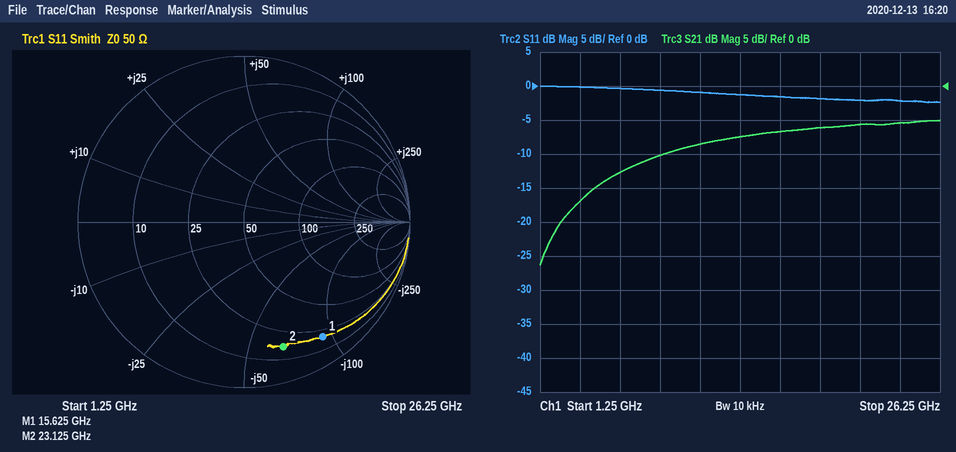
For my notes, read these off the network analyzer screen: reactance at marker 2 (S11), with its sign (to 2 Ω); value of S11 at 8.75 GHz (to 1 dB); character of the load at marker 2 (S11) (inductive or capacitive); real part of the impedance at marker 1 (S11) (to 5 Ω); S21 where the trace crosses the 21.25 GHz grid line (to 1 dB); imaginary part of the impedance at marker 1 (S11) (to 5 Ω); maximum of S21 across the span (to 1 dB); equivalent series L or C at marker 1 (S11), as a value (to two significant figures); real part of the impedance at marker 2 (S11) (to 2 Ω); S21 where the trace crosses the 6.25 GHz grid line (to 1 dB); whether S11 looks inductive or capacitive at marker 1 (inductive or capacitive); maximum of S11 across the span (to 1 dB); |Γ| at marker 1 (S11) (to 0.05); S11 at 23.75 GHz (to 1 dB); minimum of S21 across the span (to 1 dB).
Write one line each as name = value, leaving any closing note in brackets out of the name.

reactance at marker 2 (S11), with its sign = -66 Ω
value of S11 at 8.75 GHz = -1 dB
character of the load at marker 2 (S11) = capacitive
real part of the impedance at marker 1 (S11) = 20 Ω
S21 where the trace crosses the 21.25 GHz grid line = -6 dB
imaginary part of the impedance at marker 1 (S11) = -90 Ω
maximum of S21 across the span = -5 dB
equivalent series L or C at marker 1 (S11), as a value = 110 fF
real part of the impedance at marker 2 (S11) = 16 Ω
S21 where the trace crosses the 6.25 GHz grid line = -13 dB
whether S11 looks inductive or capacitive at marker 1 = capacitive
maximum of S11 across the span = 0 dB
|Γ| at marker 1 (S11) = 0.85
S11 at 23.75 GHz = -2 dB
minimum of S21 across the span = -26 dB
